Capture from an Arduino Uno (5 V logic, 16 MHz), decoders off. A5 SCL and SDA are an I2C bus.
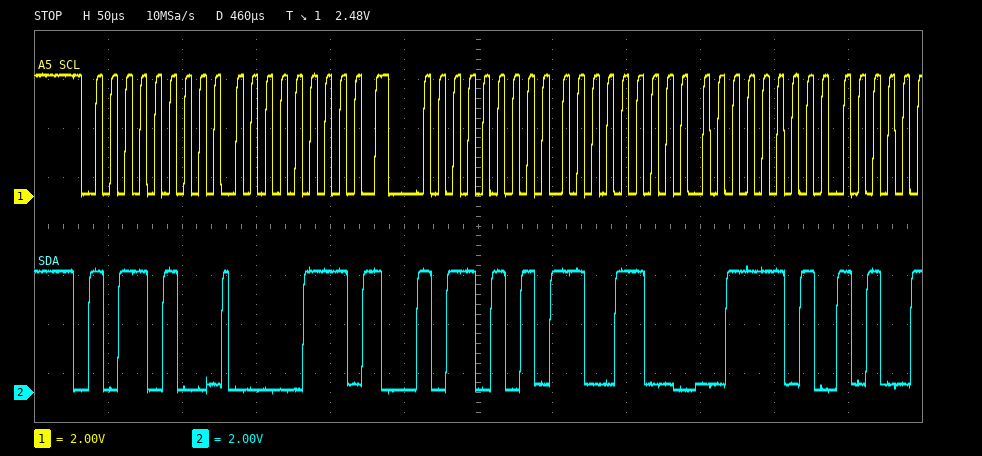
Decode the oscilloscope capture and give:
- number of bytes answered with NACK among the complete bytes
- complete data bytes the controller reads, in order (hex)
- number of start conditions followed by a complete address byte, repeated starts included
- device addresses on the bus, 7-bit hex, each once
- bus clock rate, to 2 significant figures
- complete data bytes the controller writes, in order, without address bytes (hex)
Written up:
0
CC 3D
2
0x5A
100 kHz
07
